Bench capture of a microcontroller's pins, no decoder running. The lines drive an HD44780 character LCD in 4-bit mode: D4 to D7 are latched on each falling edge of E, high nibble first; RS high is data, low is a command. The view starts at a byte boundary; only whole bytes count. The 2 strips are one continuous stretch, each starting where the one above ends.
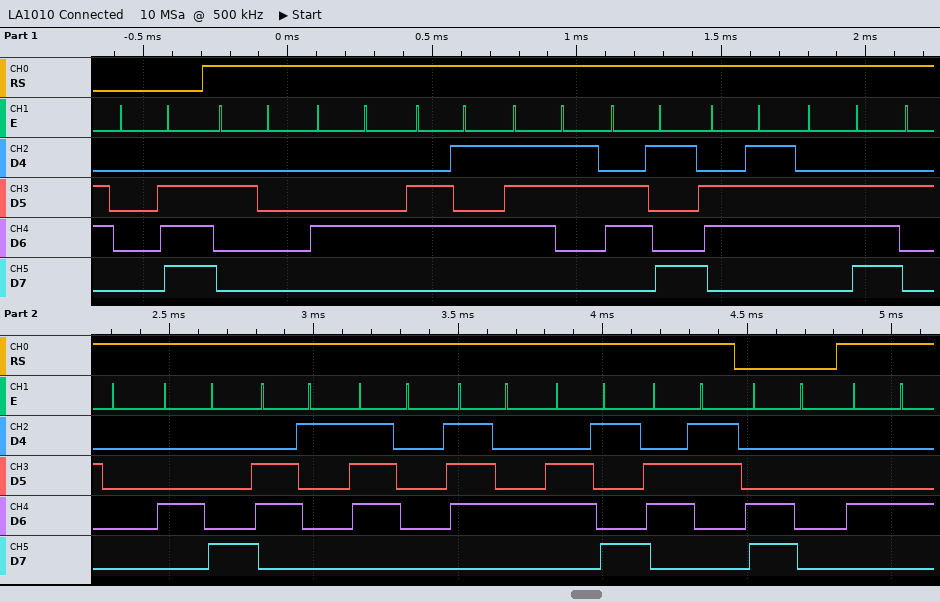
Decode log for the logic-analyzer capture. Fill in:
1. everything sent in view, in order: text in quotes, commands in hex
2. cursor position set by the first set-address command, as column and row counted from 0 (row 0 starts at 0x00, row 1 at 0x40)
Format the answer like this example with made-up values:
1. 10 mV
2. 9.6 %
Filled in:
1. 0x0E " Design Haptic" 0xC0 "D"
2. column 0, row 1
